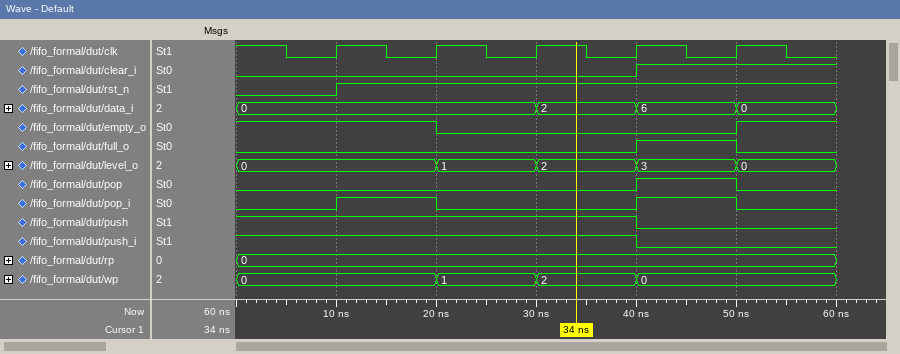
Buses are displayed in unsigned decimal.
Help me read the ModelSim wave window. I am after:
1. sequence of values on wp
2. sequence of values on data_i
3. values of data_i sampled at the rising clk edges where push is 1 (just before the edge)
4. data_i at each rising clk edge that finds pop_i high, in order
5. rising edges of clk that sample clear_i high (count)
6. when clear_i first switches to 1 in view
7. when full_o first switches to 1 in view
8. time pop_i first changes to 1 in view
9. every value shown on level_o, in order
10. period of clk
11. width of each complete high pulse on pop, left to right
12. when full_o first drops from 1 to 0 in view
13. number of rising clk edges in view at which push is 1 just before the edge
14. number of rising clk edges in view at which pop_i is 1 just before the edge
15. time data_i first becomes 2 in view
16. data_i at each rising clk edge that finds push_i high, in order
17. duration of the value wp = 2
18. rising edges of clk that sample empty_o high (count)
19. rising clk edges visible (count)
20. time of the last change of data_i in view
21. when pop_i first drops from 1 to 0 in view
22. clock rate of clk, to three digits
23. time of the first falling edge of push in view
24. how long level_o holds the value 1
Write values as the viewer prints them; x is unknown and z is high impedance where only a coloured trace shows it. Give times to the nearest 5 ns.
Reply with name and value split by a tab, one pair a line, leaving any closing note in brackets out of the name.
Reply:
sequence of values on wp	0, 1, 2, 0
sequence of values on data_i	0, 2, 6, 0
values of data_i sampled at the rising clk edges where push is 1	0, 0, 0, 2
data_i at each rising clk edge that finds pop_i high, in order	0, 6
rising edges of clk that sample clear_i high	1
when clear_i first switches to 1 in view	40 ns
when full_o first switches to 1 in view	40 ns
time pop_i first changes to 1 in view	10 ns
every value shown on level_o, in order	0, 1, 2, 3, 0
period of clk	10 ns
width of each complete high pulse on pop, left to right	10 ns
when full_o first drops from 1 to 0 in view	50 ns
number of rising clk edges in view at which push is 1 just before the edge	4
number of rising clk edges in view at which pop_i is 1 just before the edge	2
time data_i first becomes 2 in view	30 ns
data_i at each rising clk edge that finds push_i high, in order	0, 0, 0, 2
duration of the value wp = 2	10 ns
rising edges of clk that sample empty_o high	2
rising clk edges visible	5
time of the last change of data_i in view	50 ns
when pop_i first drops from 1 to 0 in view	20 ns
clock rate of clk, to three digits	100 MHz
time of the first falling edge of push in view	40 ns
how long level_o holds the value 1	10 ns
